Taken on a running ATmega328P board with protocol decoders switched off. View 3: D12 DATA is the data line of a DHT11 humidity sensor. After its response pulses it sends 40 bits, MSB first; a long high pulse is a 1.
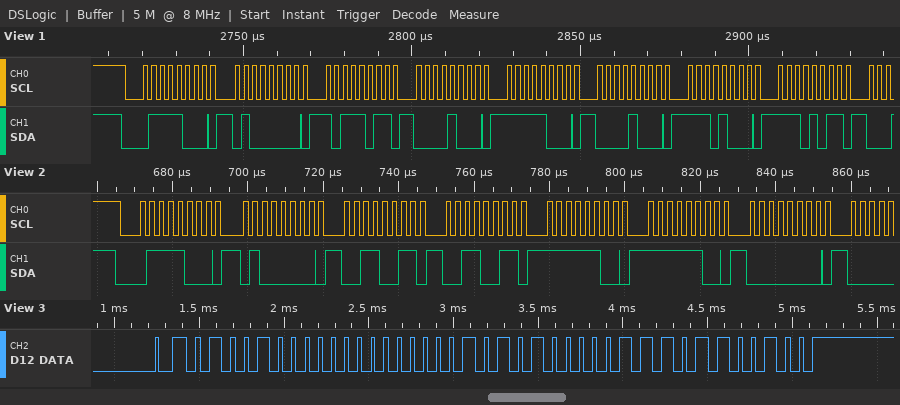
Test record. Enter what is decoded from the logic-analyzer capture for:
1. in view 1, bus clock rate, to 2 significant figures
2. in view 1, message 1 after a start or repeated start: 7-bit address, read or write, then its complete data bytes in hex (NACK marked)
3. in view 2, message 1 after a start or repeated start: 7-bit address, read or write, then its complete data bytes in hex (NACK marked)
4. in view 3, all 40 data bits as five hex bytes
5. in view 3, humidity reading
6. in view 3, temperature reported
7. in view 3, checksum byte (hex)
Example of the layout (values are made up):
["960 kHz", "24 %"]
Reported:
["400 kHz", "0x3C write: 40 BB 08 F8 08 E8 EB", "0x3C write: 40 33 33 FC FC 00", "48 00 15 07 64", "72 %", "21.7 °C", "0x64"]
